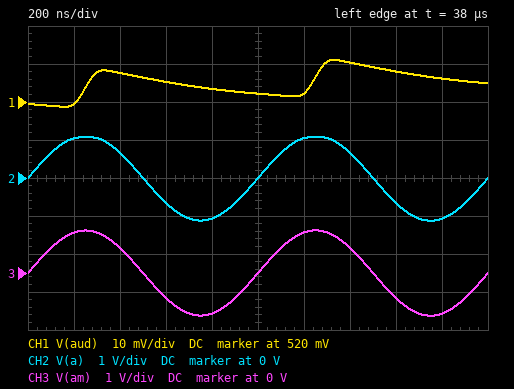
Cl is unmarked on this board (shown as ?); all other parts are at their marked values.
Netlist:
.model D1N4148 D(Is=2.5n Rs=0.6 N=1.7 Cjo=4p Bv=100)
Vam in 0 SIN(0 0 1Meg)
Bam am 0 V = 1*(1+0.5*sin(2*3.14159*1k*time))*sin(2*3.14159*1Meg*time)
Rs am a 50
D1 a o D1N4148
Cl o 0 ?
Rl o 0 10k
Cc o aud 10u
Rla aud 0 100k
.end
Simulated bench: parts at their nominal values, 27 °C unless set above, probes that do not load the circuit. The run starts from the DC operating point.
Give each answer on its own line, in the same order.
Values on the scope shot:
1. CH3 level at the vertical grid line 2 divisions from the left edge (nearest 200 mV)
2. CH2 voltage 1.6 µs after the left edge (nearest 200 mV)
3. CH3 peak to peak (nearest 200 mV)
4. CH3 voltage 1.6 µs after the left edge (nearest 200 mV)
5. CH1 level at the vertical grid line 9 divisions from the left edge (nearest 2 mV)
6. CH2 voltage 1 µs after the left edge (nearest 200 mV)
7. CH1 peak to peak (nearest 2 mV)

600 mV
-600 mV
2.2 V
-600 mV
526 mV
0 V
12 mV
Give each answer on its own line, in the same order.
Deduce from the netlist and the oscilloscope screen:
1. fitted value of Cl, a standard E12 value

6.8 nF
